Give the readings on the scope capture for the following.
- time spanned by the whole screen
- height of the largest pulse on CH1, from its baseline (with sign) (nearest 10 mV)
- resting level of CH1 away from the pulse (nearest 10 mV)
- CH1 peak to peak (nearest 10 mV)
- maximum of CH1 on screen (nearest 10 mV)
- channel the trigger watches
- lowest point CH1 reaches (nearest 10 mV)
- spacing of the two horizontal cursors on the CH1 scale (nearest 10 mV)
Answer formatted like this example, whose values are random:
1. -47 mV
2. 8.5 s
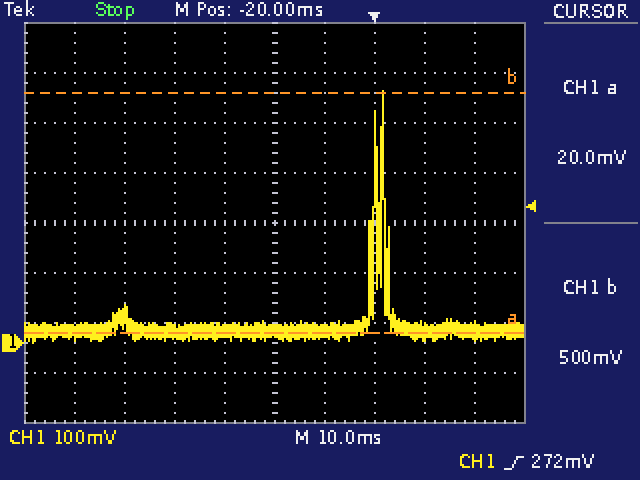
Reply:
1. 100 ms
2. +480 mV
3. 20 mV
4. 500 mV
5. 500 mV
6. CH1
7. 0 mV
8. 480 mV
